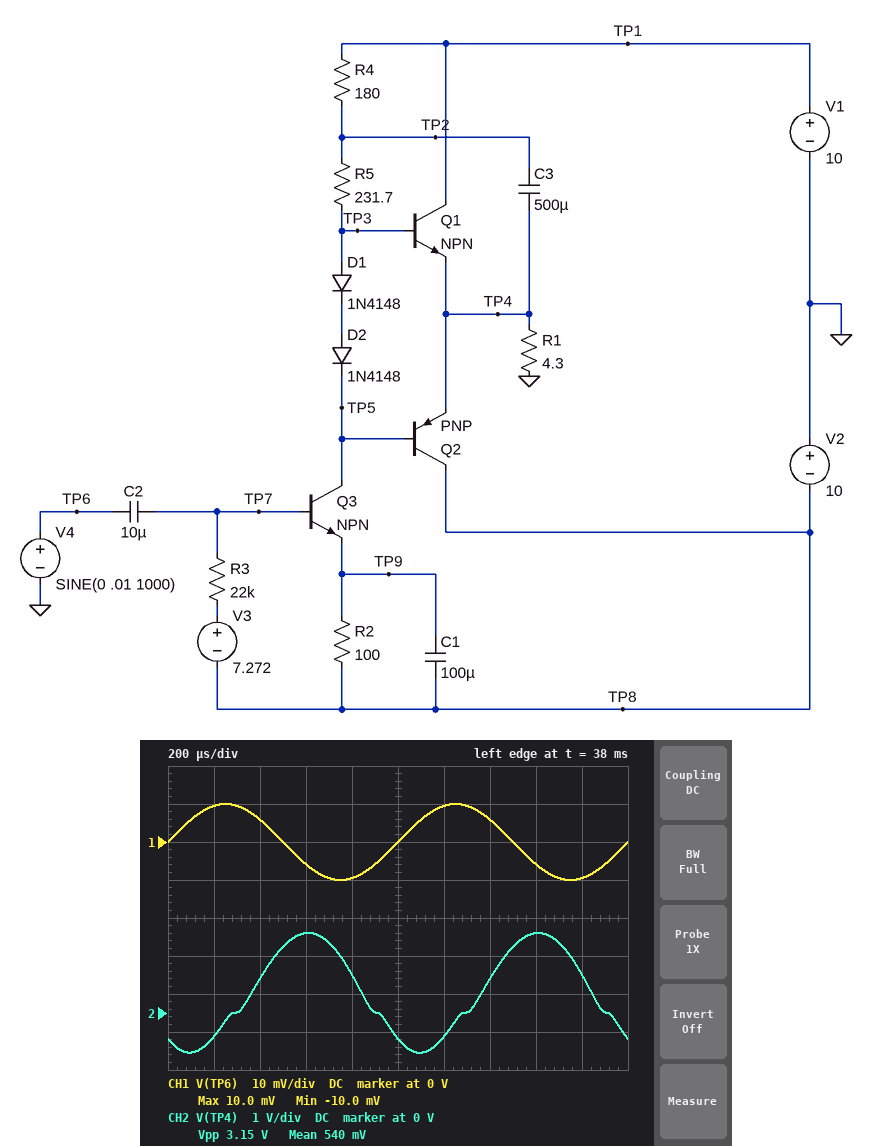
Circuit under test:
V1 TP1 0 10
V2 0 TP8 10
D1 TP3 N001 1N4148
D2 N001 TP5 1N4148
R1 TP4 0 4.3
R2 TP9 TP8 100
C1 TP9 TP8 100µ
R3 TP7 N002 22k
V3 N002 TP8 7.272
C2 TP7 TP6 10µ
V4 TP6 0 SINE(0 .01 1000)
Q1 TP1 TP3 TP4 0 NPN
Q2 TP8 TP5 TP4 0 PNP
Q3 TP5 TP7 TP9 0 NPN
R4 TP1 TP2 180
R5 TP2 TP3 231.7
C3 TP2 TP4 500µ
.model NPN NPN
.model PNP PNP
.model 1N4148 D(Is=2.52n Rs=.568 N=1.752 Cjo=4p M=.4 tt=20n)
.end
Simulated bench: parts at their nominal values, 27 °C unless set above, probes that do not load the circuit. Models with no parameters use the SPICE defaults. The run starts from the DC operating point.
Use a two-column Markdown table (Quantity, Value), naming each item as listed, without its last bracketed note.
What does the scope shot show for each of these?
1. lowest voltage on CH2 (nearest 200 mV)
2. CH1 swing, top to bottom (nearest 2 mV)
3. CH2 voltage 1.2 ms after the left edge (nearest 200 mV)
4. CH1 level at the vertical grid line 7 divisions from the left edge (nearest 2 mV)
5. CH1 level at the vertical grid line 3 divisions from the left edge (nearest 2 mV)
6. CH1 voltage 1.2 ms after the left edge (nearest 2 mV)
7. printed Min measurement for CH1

| Quantity | Value |
|---|---|
| lowest voltage on CH2 | -1.0 V |
| CH1 swing, top to bottom | 20 mV |
| CH2 voltage 1.2 ms after the left edge | -600 mV |
| CH1 level at the vertical grid line 7 divisions from the left edge | 6 mV |
| CH1 level at the vertical grid line 3 divisions from the left edge | -6 mV |
| CH1 voltage 1.2 ms after the left edge | 10 mV |
| printed Min measurement for CH1 | -10.0 mV |
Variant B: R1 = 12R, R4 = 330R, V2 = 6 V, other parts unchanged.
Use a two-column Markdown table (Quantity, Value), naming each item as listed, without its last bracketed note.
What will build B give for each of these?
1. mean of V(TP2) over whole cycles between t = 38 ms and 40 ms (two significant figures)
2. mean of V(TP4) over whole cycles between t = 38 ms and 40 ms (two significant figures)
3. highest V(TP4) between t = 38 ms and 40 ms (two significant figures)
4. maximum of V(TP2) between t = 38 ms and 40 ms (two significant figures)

| Quantity | Value |
|---|---|
| mean of V(TP2) over whole cycles between t = 38 ms and 40 ms | 4.5 V |
| mean of V(TP4) over whole cycles between t = 38 ms and 40 ms | -340 mV |
| highest V(TP4) between t = 38 ms and 40 ms | 3.1 V |
| maximum of V(TP2) between t = 38 ms and 40 ms | 7.9 V |
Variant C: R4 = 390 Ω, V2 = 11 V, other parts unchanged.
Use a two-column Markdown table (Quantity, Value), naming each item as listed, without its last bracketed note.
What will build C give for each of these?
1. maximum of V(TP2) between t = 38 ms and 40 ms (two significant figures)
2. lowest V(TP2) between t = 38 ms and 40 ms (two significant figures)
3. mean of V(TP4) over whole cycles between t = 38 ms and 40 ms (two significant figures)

| Quantity | Value |
|---|---|
| maximum of V(TP2) between t = 38 ms and 40 ms | 4.6 V |
| lowest V(TP2) between t = 38 ms and 40 ms | 1.4 V |
| mean of V(TP4) over whole cycles between t = 38 ms and 40 ms | -1.3 V |
